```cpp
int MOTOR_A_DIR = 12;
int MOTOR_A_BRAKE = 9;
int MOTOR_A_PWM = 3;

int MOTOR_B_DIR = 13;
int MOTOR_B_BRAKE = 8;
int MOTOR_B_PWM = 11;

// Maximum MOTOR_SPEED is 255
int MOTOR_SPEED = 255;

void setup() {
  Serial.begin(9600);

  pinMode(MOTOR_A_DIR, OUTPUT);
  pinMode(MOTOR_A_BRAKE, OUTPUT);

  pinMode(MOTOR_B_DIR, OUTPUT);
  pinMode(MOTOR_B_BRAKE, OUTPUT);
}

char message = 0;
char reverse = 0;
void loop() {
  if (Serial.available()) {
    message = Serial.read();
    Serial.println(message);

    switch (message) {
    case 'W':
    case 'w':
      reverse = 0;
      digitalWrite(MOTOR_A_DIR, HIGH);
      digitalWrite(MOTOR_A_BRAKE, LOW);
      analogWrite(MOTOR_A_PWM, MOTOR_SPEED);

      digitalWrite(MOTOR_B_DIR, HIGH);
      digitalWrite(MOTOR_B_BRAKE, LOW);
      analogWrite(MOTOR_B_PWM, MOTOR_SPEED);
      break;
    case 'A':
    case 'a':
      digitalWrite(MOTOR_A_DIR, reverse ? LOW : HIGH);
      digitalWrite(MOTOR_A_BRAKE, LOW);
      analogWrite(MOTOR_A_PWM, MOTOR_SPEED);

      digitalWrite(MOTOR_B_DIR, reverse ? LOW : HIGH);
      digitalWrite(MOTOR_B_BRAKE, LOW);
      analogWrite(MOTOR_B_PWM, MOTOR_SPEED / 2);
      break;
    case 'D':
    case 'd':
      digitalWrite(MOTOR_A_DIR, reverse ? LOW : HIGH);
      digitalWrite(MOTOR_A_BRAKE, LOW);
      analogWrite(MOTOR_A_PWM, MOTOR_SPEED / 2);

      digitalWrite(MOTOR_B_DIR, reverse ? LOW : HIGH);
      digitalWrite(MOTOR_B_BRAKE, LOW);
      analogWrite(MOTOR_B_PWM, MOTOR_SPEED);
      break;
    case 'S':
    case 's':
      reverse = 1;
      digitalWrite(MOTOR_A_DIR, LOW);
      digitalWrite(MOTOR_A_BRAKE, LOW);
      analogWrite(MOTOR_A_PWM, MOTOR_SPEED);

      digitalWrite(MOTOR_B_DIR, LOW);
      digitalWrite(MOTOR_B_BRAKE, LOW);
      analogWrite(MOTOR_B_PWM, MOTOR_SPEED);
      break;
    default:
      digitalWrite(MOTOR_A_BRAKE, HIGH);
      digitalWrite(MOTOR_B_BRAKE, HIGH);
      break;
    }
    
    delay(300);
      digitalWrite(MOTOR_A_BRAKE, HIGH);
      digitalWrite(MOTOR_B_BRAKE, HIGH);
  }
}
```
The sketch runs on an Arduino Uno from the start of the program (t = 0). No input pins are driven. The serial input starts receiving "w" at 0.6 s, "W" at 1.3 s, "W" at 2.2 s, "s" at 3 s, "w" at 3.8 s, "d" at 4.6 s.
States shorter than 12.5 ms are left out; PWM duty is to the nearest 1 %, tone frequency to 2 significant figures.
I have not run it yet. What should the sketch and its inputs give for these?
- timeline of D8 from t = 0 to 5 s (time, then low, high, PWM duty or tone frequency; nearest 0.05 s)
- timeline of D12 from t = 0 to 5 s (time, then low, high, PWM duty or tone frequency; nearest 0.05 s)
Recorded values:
0 s low; 0.9 s high; 1.3 s low; 1.6 s high; 2.2 s low; 2.5 s high; 3 s low; 3.3 s high; 3.8 s low; 4.1 s high; 4.6 s low; 4.9 s high
0 s low; 0.6 s high; 3 s low; 3.8 s high
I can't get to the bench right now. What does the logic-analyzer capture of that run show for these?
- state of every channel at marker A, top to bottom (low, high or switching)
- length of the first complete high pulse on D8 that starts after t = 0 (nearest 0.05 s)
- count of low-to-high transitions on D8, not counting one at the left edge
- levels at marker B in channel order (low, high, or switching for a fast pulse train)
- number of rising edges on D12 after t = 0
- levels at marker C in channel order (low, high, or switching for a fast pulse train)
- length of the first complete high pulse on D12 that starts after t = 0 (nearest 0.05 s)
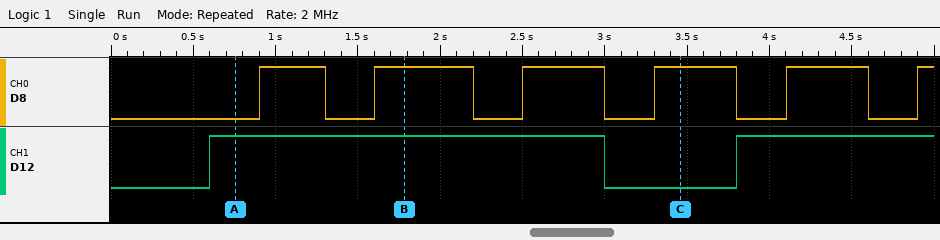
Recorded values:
D8 low, D12 high
0.40 s
6
D8 high, D12 high
2
D8 high, D12 low
2.40 s
